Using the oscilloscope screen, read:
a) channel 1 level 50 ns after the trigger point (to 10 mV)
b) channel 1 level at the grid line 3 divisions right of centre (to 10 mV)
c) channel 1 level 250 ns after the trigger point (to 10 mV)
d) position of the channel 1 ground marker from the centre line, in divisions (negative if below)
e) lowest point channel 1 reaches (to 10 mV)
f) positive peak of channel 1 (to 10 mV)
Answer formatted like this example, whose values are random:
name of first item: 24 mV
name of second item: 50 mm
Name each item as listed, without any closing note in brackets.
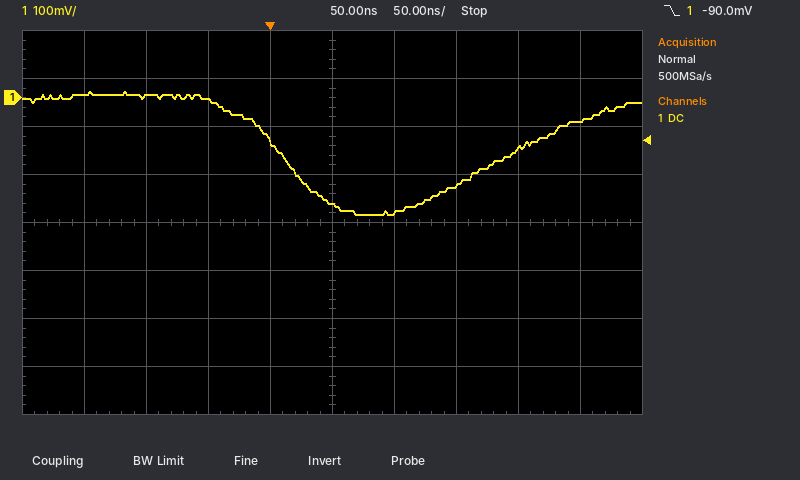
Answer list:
channel 1 level 50 ns after the trigger point: -220 mV
channel 1 level at the grid line 3 divisions right of centre: -110 mV
channel 1 level 250 ns after the trigger point: -50 mV
position of the channel 1 ground marker from the centre line, in divisions: +2.6 div
lowest point channel 1 reaches: -240 mV
positive peak of channel 1: 10 mV
